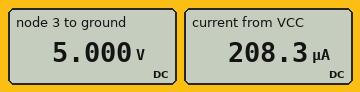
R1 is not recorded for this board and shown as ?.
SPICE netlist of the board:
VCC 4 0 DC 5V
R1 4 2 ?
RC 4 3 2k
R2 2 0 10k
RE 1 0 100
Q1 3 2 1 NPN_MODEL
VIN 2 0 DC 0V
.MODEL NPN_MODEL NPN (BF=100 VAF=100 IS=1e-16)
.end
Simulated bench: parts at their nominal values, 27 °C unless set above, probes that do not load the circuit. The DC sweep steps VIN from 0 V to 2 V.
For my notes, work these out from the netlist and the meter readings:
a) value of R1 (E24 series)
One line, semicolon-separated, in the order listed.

24 kΩ
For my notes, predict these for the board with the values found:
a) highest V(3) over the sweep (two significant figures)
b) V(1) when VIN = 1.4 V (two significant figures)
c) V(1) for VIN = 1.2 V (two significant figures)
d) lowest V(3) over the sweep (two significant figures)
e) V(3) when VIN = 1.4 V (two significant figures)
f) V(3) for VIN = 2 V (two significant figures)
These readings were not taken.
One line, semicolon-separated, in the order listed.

5.0 V; 570 mV; 380 mV; 320 mV; 590 mV; 1.2 V
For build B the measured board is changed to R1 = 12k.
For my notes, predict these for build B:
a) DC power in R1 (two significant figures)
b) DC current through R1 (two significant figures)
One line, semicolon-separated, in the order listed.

2.1 mW; 420 µA
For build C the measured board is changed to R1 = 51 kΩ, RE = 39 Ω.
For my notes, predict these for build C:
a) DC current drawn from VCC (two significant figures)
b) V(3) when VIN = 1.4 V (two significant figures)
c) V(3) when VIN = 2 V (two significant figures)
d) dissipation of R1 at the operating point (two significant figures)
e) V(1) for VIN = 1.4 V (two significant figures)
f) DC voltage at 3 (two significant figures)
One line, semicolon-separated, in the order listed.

98 µA; 560 mV; 1.1 V; 490 µW; 540 mV; 5.0 V
